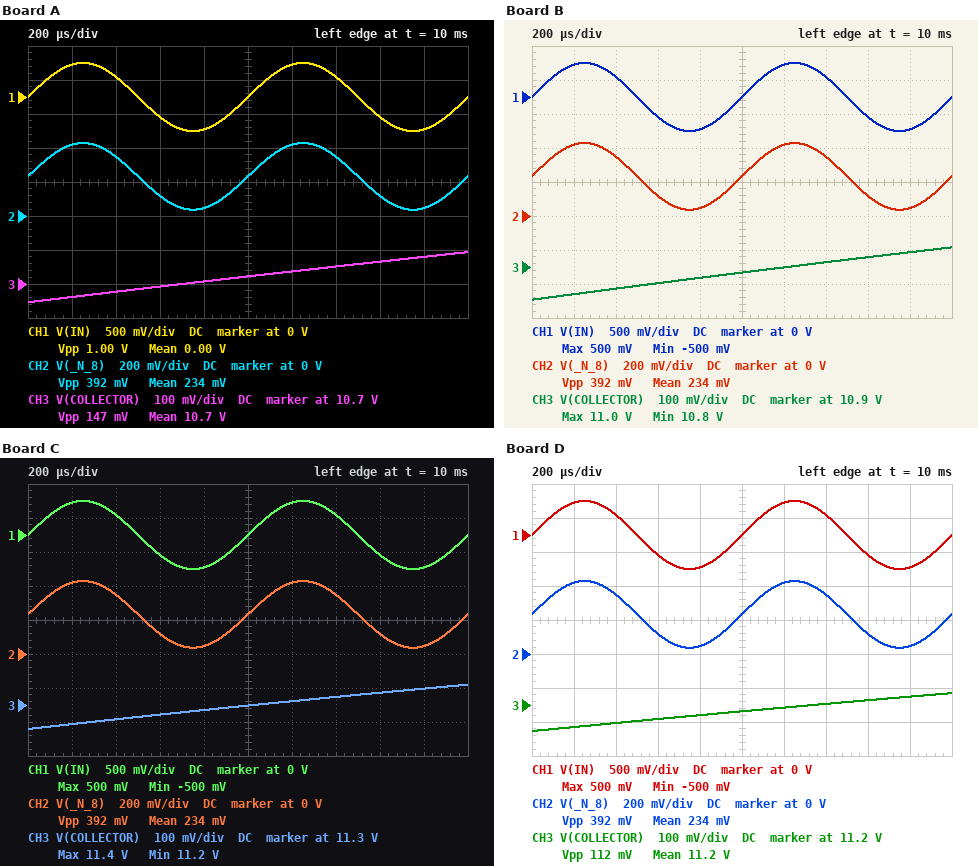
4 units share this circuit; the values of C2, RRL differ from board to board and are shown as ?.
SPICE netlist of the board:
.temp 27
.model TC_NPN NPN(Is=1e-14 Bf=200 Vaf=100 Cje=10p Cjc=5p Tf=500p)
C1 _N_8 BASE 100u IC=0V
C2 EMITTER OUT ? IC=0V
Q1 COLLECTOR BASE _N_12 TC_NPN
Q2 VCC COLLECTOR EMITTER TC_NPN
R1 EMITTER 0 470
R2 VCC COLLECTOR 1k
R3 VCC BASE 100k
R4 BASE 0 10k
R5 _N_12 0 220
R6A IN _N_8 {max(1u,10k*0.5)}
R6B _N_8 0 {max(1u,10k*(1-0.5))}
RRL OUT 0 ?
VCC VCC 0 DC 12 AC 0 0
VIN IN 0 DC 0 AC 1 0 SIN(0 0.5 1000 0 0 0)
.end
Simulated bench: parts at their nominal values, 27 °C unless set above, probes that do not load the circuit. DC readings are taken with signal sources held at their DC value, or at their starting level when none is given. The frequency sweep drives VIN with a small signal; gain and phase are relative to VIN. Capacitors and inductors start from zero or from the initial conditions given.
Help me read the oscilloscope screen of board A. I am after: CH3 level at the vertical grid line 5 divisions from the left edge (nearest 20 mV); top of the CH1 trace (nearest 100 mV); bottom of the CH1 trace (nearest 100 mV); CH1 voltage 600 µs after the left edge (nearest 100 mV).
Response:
10.72 V
500 mV
-500 mV
-300 mV
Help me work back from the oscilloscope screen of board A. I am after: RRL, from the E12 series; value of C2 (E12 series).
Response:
18 Ω
680 µF
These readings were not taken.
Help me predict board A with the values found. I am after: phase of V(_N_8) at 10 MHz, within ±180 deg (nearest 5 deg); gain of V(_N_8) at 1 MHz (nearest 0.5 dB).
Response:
-30 deg
-8.5 dB
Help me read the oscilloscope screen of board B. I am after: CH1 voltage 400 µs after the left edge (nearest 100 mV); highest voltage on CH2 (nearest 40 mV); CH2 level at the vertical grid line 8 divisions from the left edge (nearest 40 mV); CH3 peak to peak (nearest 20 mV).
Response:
300 mV
440 mV
120 mV
160 mV
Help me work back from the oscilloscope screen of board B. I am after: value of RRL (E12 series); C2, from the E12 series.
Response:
18 Ω
560 µF
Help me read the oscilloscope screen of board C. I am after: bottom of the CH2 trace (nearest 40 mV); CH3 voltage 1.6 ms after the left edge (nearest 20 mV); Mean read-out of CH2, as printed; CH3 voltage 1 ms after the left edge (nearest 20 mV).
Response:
40 mV
11.34 V
234 mV
11.30 V
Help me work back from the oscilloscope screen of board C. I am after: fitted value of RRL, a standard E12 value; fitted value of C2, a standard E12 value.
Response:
22 Ω
330 µF
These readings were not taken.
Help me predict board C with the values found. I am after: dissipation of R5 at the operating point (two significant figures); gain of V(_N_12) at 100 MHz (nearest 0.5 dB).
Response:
580 µW
-25.0 dB
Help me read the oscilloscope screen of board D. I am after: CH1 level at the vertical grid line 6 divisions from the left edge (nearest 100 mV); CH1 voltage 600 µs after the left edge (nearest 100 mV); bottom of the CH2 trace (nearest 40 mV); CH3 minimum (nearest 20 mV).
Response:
500 mV
-300 mV
40 mV
11.12 V
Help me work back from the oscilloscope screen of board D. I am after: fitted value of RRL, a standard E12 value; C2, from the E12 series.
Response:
27 Ω
390 µF
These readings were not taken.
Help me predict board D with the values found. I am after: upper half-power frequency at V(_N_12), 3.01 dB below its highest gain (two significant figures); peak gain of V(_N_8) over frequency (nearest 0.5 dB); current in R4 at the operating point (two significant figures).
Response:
5.5 MHz
-8.5 dB
100 µA
